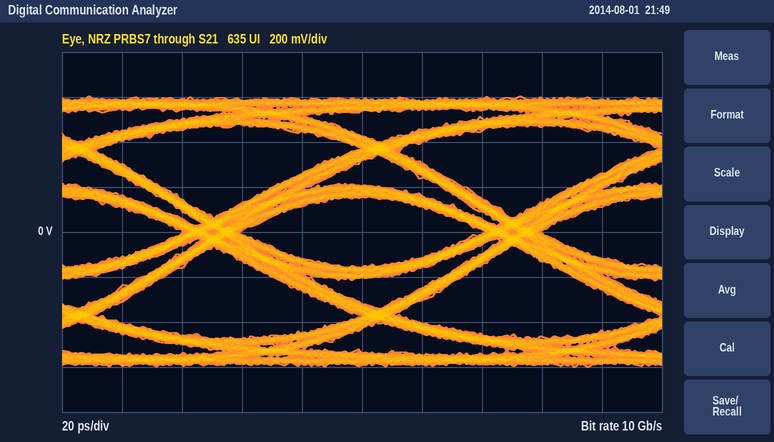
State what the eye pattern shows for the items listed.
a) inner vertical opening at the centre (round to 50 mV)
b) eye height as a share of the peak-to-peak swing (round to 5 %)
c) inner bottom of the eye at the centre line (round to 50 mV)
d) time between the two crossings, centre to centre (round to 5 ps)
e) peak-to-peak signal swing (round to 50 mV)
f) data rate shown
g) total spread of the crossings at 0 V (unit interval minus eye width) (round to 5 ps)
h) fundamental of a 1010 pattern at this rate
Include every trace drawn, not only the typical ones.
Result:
300 mV
25 %
-150 mV
100 ps
1.20 V
10 Gb/s
20 ps
5 GHz
